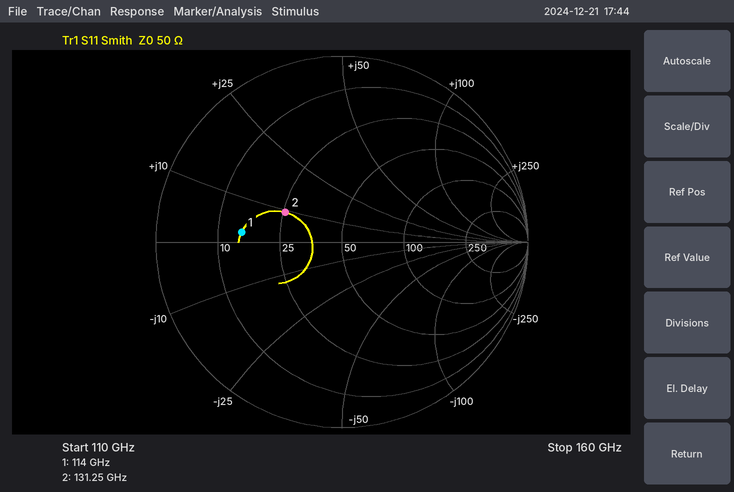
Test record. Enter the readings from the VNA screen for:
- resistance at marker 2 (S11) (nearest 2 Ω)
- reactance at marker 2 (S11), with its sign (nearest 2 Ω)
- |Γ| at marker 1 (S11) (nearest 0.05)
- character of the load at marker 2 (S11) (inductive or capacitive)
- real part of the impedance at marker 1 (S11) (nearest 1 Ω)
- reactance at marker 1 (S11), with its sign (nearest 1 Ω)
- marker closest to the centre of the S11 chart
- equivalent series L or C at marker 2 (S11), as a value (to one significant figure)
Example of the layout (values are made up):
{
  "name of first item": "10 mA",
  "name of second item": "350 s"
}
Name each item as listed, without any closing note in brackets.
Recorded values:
{
  "resistance at marker 2 (S11)": "26 Ω",
  "reactance at marker 2 (S11), with its sign": "+10 Ω",
  "|Γ| at marker 1 (S11)": "0.55",
  "character of the load at marker 2 (S11)": "inductive",
  "real part of the impedance at marker 1 (S11)": "15 Ω",
  "reactance at marker 1 (S11), with its sign": "+2 Ω",
  "marker closest to the centre of the S11 chart": "marker 2",
  "equivalent series L or C at marker 2 (S11), as a value": "10 pH"
}
